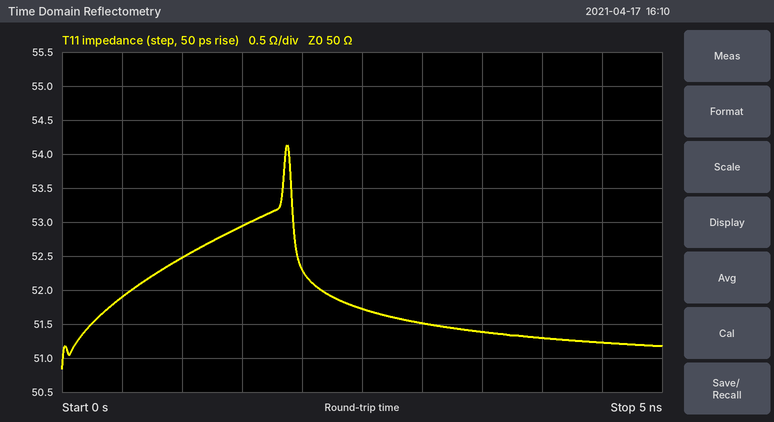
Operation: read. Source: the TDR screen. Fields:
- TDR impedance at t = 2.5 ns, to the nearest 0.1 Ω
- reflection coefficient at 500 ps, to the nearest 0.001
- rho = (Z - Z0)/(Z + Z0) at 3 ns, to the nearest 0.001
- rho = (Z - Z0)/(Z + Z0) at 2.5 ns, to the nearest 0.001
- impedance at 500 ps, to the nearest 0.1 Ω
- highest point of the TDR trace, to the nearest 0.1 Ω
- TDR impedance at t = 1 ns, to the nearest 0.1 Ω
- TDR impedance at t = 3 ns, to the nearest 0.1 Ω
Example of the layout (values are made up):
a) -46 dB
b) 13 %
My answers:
a) 51.7 Ω
b) +0.019
c) +0.015
d) +0.017
e) 51.9 Ω
f) 54.1 Ω
g) 52.5 Ω
h) 51.5 Ω
